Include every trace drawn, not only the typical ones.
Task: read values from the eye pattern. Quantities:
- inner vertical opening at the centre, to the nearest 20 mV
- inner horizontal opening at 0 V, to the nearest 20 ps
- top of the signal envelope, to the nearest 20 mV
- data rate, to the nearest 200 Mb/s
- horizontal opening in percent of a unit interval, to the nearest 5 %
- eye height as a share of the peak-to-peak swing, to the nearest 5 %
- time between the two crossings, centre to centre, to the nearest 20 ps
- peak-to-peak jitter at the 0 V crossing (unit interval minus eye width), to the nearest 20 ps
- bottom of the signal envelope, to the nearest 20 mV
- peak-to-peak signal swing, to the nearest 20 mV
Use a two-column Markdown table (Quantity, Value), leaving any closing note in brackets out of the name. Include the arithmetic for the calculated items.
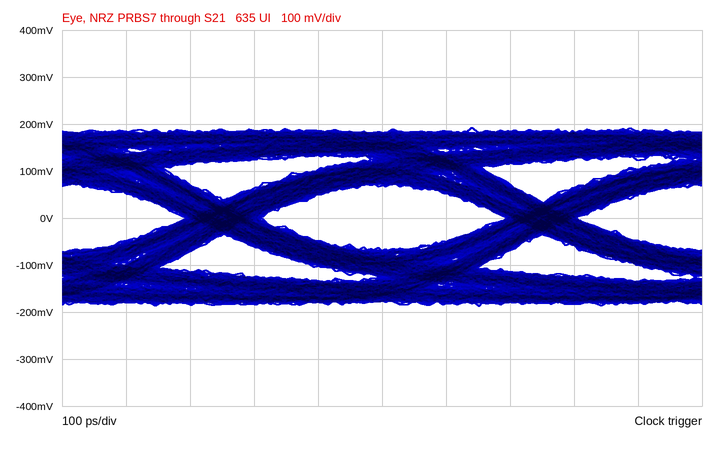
| Quantity | Value |
|---|---|
| inner vertical opening at the centre, to the nearest 20 mV | 140 mV |
| inner horizontal opening at 0 V, to the nearest 20 ps | 380 ps |
| top of the signal envelope, to the nearest 20 mV | 200 mV |
| data rate, to the nearest 200 Mb/s | 2.0 Gb/s |
| horizontal opening in percent of a unit interval, to the nearest 5 % | 380 ps / 500 ps ≈ 76.0 %, so 75 % to the nearest 5 % |
| eye height as a share of the peak-to-peak swing, to the nearest 5 % | 140 mV / 380 mV ≈ 36.8 %, so 35 % to the nearest 5 % |
| time between the two crossings, centre to centre, to the nearest 20 ps | 500 ps |
| peak-to-peak jitter at the 0 V crossing (unit interval minus eye width), to the nearest 20 ps | 120 ps |
| bottom of the signal envelope, to the nearest 20 mV | -180 mV |
| peak-to-peak signal swing, to the nearest 20 mV | 380 mV |
